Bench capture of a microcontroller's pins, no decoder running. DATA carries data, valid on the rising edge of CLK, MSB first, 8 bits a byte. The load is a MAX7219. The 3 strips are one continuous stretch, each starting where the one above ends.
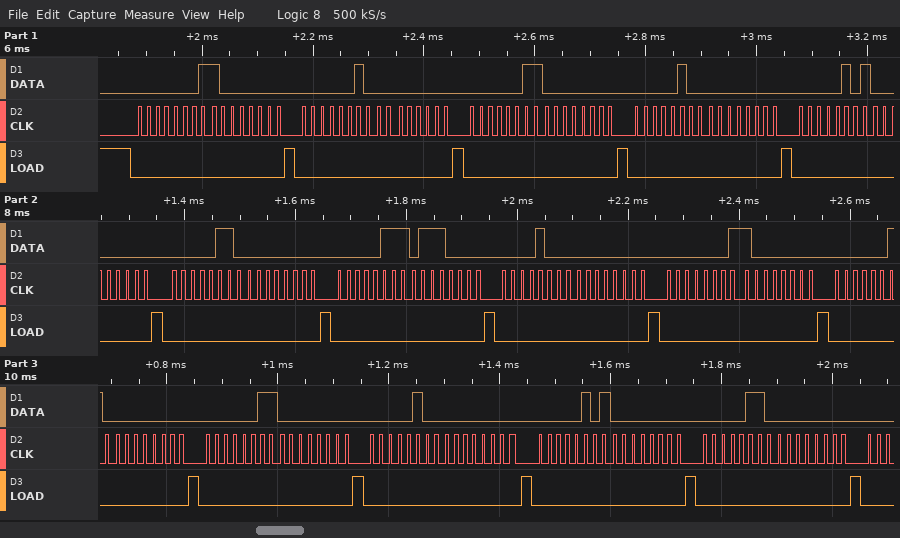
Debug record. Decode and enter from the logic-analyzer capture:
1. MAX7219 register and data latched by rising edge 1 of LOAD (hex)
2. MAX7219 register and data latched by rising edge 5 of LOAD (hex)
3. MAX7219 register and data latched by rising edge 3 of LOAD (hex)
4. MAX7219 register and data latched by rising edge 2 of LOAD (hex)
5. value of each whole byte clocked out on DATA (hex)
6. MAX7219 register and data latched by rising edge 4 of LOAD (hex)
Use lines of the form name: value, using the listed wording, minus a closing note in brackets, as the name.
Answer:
MAX7219 register and data latched by rising edge 1 of LOAD: register 0x1, data 0x80
MAX7219 register and data latched by rising edge 5 of LOAD: register 0x5, data 0x00
MAX7219 register and data latched by rising edge 3 of LOAD: register 0x3, data 0x00
MAX7219 register and data latched by rising edge 2 of LOAD: register 0x2, data 0x00
value of each whole byte clocked out on DATA: 01 80 02 00 03 00 04 00 05 00 06 00 07 70 08 00 01 80 02 00 03 00 04 00 05 00 06 00
MAX7219 register and data latched by rising edge 4 of LOAD: register 0x4, data 0x00
